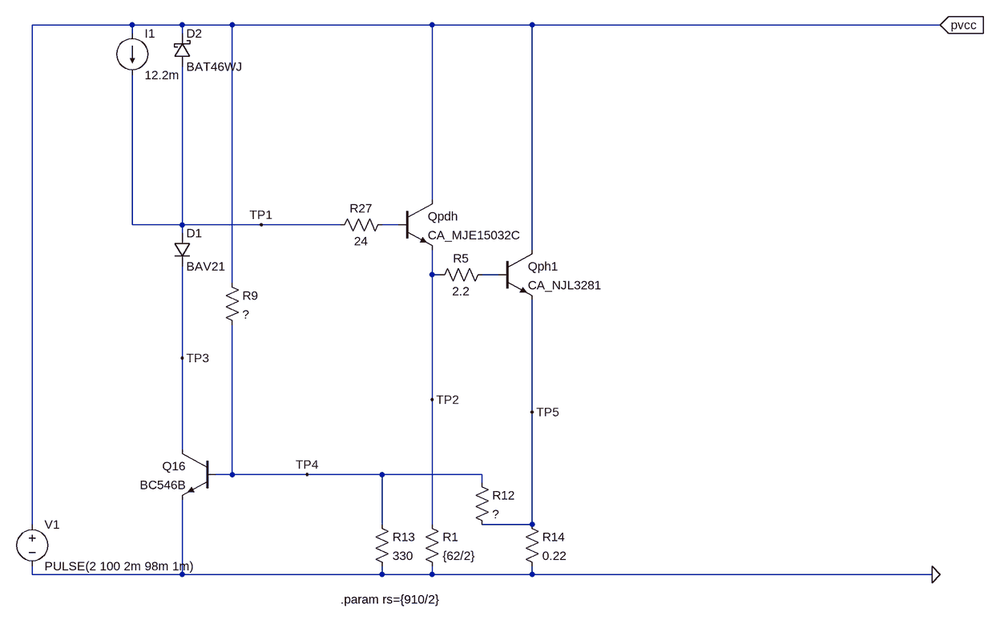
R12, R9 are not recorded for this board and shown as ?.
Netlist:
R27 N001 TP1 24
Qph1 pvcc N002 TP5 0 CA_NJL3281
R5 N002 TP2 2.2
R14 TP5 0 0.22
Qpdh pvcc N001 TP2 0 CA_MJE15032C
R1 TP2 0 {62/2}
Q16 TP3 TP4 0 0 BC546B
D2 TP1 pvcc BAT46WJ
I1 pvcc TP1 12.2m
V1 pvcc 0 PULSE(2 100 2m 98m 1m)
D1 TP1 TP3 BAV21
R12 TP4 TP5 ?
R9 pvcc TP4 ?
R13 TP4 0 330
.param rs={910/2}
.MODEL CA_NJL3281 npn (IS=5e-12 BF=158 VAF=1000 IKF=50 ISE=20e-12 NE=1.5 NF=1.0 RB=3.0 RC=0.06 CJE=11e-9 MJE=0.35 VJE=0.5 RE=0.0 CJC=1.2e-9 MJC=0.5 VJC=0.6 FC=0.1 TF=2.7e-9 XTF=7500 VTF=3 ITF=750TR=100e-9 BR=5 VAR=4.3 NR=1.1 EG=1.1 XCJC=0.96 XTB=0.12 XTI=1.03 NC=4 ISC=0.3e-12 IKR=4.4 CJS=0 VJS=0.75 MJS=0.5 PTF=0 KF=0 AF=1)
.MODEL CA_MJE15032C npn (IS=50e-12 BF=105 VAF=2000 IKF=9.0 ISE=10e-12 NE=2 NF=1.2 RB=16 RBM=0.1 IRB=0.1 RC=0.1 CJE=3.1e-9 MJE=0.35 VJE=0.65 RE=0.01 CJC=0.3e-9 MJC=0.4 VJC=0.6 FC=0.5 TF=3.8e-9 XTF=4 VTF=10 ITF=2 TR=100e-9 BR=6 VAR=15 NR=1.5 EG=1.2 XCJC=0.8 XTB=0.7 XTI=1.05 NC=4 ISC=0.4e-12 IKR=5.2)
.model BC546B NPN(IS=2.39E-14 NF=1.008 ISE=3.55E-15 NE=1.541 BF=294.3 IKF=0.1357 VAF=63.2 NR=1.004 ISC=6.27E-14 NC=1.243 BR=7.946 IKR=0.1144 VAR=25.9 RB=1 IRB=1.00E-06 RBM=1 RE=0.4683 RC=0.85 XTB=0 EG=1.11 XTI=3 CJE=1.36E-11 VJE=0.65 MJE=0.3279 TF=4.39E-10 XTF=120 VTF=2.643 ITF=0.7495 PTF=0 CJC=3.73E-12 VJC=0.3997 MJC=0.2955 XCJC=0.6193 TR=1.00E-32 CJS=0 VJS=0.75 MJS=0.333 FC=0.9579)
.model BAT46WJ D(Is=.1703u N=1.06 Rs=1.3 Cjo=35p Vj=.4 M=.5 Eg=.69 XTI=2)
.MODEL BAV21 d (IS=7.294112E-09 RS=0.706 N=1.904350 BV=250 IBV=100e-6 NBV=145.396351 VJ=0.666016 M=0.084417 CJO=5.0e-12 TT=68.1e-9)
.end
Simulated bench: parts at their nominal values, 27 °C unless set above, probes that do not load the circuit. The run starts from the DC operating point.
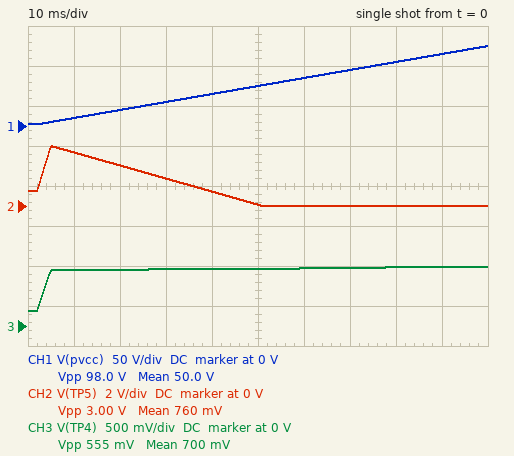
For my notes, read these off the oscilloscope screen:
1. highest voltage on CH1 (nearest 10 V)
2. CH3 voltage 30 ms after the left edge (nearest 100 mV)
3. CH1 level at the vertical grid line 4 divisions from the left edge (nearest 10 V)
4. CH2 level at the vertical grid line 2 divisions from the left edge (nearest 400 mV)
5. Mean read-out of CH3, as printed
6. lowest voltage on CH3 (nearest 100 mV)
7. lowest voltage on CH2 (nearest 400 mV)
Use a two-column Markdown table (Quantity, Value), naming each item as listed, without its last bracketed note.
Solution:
| Quantity | Value |
|---|---|
| highest voltage on CH1 | 100 V |
| CH3 voltage 30 ms after the left edge | 700 mV |
| CH1 level at the vertical grid line 4 divisions from the left edge | 40 V |
| CH2 level at the vertical grid line 2 divisions from the left edge | 2.0 V |
| Mean read-out of CH3, as printed | 700 mV |
| lowest voltage on CH3 | 200 mV |
| lowest voltage on CH2 | 0 V |
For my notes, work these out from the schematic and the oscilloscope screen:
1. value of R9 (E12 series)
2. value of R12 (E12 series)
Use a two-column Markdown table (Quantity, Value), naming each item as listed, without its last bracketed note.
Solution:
| Quantity | Value |
|---|---|
| value of R9 | 18 kΩ |
| value of R12 | 1.2 kΩ |
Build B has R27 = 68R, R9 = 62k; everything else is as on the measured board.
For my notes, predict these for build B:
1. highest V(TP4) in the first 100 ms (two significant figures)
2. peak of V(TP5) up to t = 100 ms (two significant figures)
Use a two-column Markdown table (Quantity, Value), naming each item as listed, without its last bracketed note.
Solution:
| Quantity | Value |
|---|---|
| highest V(TP4) in the first 100 ms | 710 mV |
| peak of V(TP5) up to t = 100 ms | 3.2 V |
